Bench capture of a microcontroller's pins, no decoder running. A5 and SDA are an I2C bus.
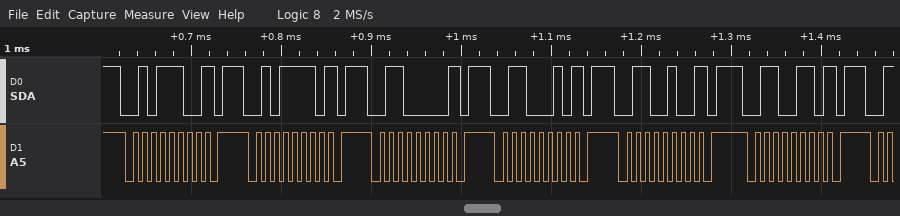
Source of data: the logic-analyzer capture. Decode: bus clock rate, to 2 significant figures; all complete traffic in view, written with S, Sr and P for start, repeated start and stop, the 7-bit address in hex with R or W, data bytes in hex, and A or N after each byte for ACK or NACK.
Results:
100 kHz
S 2EW N P S 2FW N P S 30W N P S 31W N P S 32W N P S 33W N P
